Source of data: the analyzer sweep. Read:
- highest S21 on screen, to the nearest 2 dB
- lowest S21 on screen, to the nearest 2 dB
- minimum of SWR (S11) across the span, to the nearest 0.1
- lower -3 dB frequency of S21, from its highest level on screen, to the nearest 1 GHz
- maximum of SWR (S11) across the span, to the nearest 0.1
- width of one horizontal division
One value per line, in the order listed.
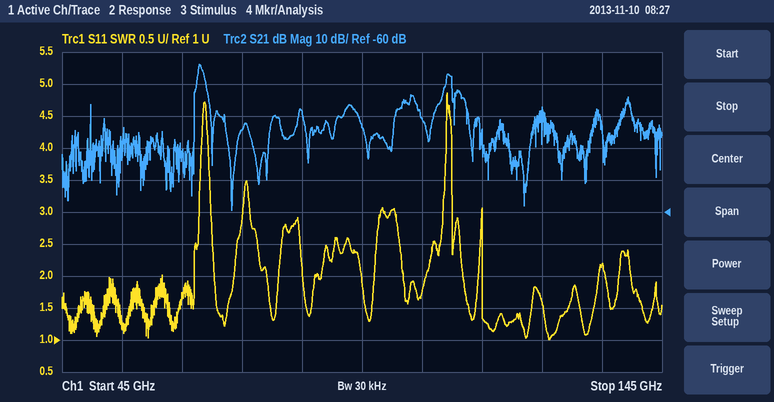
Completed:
-14 dB
-60 dB
1.0
68 GHz
4.9
10 GHz
